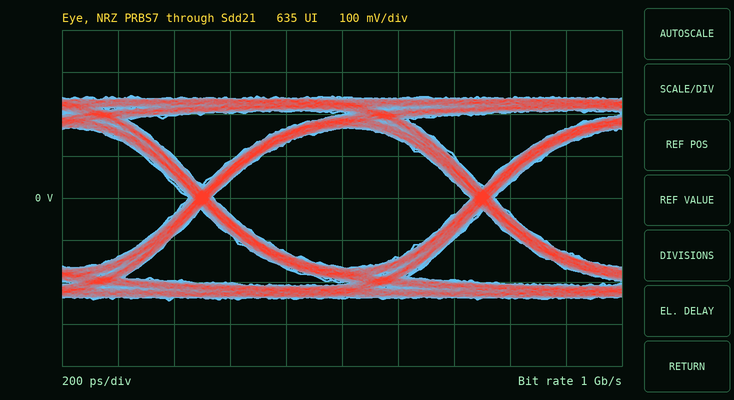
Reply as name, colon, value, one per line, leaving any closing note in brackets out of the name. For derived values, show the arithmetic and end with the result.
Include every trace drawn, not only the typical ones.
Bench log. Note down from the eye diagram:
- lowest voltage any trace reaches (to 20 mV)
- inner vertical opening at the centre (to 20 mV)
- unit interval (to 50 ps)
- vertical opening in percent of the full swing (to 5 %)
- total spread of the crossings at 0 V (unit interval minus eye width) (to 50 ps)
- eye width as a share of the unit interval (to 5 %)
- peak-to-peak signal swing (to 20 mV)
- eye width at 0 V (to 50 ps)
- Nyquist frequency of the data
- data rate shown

lowest voltage any trace reaches: -240 mV
inner vertical opening at the centre: 340 mV
unit interval: 1.00 ns
vertical opening in percent of the full swing: 340 mV / 480 mV ≈ 70.8 %, so 70 % to the nearest 5 %
total spread of the crossings at 0 V (unit interval minus eye width): 100 ps
eye width as a share of the unit interval: 900 ps / 1.00 ns ≈ 90 %
peak-to-peak signal swing: 480 mV
eye width at 0 V: 900 ps
Nyquist frequency of the data: 500 MHz
data rate shown: 1 Gb/s
